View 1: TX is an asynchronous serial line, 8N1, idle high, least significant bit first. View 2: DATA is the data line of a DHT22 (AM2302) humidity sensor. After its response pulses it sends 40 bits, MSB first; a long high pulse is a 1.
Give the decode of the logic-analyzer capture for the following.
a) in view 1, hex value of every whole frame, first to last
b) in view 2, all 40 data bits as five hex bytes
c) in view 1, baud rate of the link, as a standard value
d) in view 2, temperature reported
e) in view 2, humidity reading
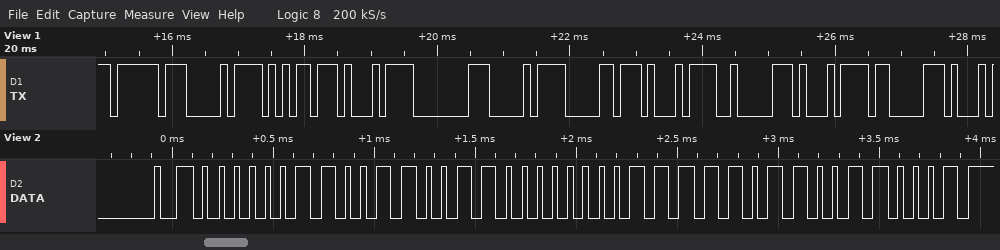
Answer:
0xBF 0xD0 0xB5 0xD1 0x80 0xD0 0xB0 0xD1 0x82 0xD1 0x83
03 33 00 FB 31
9600 baud
25.1 °C
81.9 %
